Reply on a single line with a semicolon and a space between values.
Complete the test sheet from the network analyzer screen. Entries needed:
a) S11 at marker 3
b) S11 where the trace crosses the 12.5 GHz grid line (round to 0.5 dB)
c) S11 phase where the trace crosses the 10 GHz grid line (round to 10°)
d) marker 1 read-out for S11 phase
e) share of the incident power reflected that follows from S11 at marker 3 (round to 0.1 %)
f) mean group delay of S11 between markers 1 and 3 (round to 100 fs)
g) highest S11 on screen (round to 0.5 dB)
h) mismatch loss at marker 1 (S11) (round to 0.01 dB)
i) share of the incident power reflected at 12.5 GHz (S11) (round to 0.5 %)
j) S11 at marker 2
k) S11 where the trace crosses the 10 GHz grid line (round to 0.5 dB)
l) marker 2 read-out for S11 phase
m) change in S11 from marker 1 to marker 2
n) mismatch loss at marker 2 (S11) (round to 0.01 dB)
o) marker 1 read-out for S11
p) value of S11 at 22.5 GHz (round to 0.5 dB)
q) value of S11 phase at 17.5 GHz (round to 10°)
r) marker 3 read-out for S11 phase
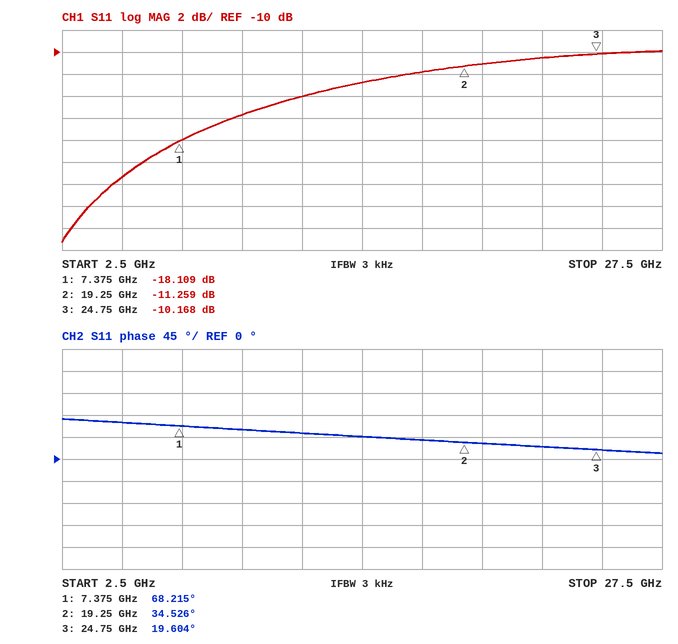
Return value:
-10.168 dB; -14.0 dB; 60°; 68.215°; 9.6 %; 7.8 ps; -10.0 dB; 0.07 dB; 4.0 %; -11.259 dB; -15.5 dB; 34.526°; 6.850 dB; 0.34 dB; -18.109 dB; -10.5 dB; 40°; 19.604°
